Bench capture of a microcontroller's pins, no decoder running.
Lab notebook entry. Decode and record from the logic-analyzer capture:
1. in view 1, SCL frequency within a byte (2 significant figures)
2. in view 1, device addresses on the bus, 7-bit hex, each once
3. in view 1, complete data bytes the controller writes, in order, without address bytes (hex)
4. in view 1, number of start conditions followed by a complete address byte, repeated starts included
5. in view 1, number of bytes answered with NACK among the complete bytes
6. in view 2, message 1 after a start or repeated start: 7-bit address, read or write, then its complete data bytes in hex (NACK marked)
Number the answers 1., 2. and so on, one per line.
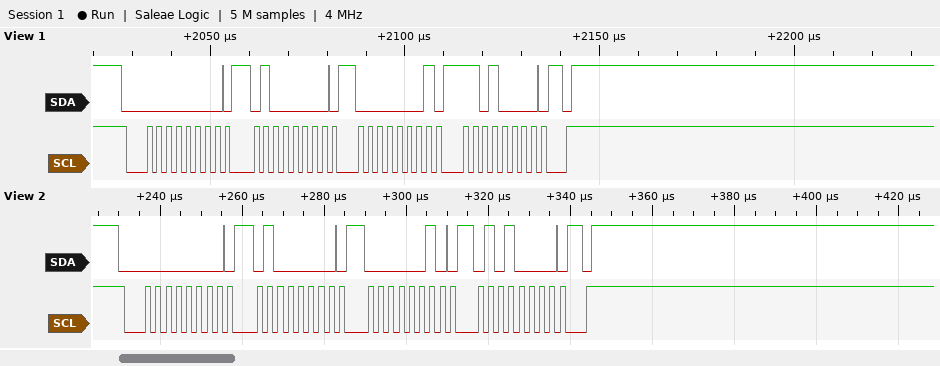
1. 400 kHz
2. 0x00
3. 40 01 D0
4. 1
5. 0
6. 0x00 write: 40 02 50
